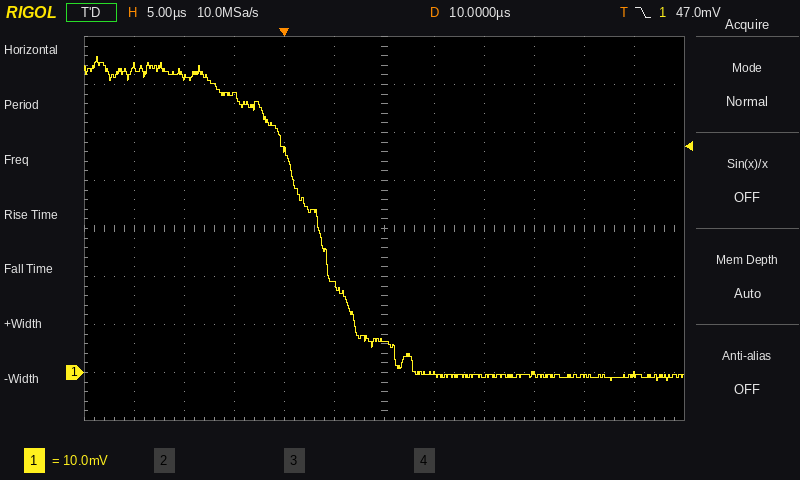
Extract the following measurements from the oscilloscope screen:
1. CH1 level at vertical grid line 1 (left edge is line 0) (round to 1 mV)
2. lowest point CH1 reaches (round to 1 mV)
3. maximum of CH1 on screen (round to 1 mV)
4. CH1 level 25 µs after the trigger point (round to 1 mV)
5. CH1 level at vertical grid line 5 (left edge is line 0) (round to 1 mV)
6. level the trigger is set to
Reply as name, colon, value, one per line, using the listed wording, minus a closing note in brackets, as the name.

CH1 level at vertical grid line 1 (left edge is line 0): 64 mV
lowest point CH1 reaches: -2 mV
maximum of CH1 on screen: 66 mV
CH1 level 25 µs after the trigger point: 0 mV
CH1 level at vertical grid line 5 (left edge is line 0): 18 mV
level the trigger is set to: 47.0 mV
